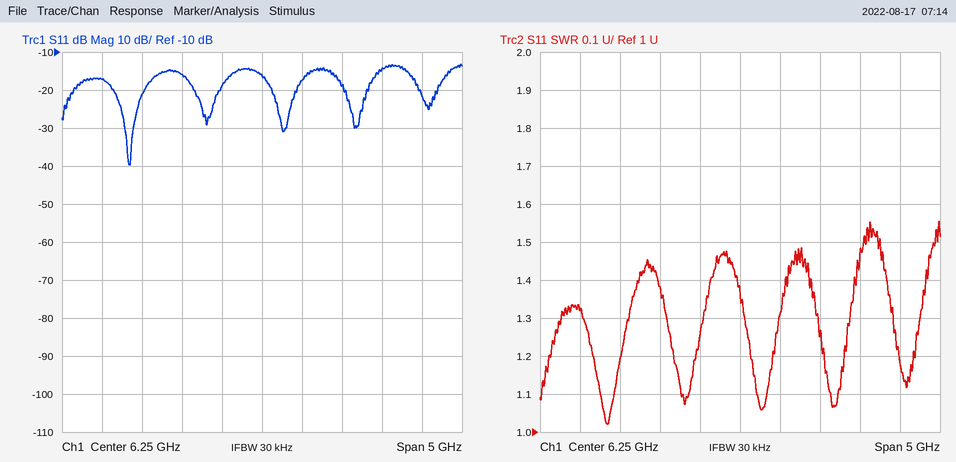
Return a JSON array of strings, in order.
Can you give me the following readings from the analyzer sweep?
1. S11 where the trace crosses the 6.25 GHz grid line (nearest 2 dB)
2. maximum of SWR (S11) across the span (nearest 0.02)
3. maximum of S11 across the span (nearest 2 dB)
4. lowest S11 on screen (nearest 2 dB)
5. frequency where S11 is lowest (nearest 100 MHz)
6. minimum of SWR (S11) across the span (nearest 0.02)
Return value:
["-16 dB", "1.56", "-14 dB", "-40 dB", "4.6 GHz", "1.02"]
